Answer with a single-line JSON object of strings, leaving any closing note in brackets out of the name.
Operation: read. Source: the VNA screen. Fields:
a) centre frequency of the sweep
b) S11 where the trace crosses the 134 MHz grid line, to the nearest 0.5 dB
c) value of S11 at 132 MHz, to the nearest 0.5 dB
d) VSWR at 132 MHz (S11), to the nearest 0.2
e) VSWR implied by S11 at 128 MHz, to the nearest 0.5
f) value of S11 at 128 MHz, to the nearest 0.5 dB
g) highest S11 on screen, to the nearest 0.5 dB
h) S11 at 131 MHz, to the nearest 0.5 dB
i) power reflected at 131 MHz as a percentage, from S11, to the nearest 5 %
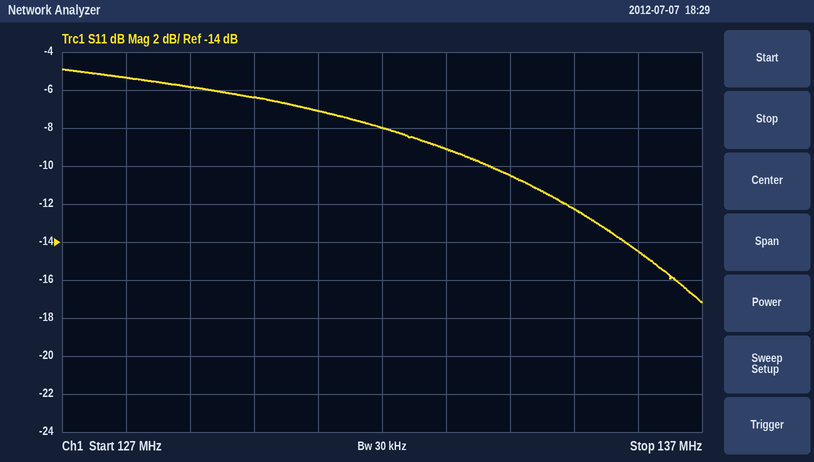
{"centre frequency of the sweep": "132 MHz", "S11 where the trace crosses the 134 MHz grid line, to the nearest 0.5 dB": "-10.5 dB", "value of S11 at 132 MHz, to the nearest 0.5 dB": "-8.0 dB", "VSWR at 132 MHz (S11), to the nearest 0.2": "2.4", "VSWR implied by S11 at 128 MHz, to the nearest 0.5": "3.5", "value of S11 at 128 MHz, to the nearest 0.5 dB": "-5.5 dB", "highest S11 on screen, to the nearest 0.5 dB": "-5.0 dB", "S11 at 131 MHz, to the nearest 0.5 dB": "-7.0 dB", "power reflected at 131 MHz as a percentage, from S11, to the nearest 5 %": "20 %"}
